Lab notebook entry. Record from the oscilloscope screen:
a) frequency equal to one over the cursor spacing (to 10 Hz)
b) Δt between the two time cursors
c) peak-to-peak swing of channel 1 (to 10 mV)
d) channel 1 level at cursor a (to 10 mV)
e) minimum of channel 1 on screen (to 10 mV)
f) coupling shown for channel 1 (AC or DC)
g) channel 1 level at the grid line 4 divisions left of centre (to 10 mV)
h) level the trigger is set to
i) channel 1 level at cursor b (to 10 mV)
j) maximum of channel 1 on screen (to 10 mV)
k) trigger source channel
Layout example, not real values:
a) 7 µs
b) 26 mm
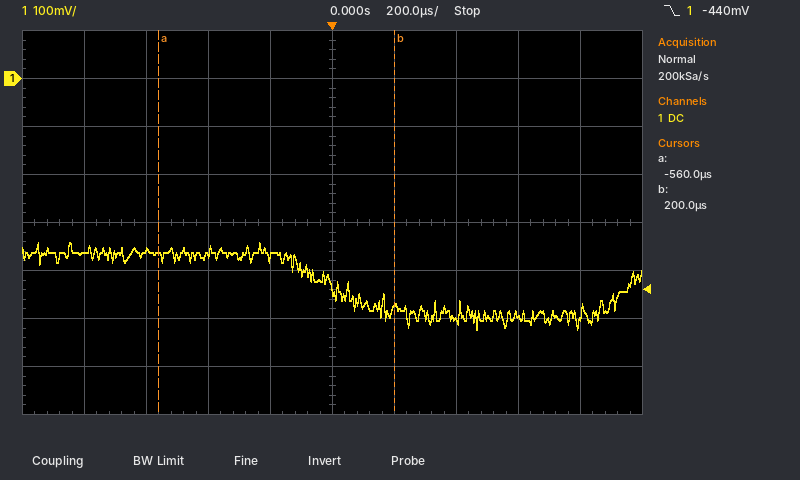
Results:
a) 1.32 kHz
b) 760 µs
c) 180 mV
d) -370 mV
e) -520 mV
f) DC
g) -360 mV
h) -440 mV
i) -480 mV
j) -340 mV
k) channel 1
